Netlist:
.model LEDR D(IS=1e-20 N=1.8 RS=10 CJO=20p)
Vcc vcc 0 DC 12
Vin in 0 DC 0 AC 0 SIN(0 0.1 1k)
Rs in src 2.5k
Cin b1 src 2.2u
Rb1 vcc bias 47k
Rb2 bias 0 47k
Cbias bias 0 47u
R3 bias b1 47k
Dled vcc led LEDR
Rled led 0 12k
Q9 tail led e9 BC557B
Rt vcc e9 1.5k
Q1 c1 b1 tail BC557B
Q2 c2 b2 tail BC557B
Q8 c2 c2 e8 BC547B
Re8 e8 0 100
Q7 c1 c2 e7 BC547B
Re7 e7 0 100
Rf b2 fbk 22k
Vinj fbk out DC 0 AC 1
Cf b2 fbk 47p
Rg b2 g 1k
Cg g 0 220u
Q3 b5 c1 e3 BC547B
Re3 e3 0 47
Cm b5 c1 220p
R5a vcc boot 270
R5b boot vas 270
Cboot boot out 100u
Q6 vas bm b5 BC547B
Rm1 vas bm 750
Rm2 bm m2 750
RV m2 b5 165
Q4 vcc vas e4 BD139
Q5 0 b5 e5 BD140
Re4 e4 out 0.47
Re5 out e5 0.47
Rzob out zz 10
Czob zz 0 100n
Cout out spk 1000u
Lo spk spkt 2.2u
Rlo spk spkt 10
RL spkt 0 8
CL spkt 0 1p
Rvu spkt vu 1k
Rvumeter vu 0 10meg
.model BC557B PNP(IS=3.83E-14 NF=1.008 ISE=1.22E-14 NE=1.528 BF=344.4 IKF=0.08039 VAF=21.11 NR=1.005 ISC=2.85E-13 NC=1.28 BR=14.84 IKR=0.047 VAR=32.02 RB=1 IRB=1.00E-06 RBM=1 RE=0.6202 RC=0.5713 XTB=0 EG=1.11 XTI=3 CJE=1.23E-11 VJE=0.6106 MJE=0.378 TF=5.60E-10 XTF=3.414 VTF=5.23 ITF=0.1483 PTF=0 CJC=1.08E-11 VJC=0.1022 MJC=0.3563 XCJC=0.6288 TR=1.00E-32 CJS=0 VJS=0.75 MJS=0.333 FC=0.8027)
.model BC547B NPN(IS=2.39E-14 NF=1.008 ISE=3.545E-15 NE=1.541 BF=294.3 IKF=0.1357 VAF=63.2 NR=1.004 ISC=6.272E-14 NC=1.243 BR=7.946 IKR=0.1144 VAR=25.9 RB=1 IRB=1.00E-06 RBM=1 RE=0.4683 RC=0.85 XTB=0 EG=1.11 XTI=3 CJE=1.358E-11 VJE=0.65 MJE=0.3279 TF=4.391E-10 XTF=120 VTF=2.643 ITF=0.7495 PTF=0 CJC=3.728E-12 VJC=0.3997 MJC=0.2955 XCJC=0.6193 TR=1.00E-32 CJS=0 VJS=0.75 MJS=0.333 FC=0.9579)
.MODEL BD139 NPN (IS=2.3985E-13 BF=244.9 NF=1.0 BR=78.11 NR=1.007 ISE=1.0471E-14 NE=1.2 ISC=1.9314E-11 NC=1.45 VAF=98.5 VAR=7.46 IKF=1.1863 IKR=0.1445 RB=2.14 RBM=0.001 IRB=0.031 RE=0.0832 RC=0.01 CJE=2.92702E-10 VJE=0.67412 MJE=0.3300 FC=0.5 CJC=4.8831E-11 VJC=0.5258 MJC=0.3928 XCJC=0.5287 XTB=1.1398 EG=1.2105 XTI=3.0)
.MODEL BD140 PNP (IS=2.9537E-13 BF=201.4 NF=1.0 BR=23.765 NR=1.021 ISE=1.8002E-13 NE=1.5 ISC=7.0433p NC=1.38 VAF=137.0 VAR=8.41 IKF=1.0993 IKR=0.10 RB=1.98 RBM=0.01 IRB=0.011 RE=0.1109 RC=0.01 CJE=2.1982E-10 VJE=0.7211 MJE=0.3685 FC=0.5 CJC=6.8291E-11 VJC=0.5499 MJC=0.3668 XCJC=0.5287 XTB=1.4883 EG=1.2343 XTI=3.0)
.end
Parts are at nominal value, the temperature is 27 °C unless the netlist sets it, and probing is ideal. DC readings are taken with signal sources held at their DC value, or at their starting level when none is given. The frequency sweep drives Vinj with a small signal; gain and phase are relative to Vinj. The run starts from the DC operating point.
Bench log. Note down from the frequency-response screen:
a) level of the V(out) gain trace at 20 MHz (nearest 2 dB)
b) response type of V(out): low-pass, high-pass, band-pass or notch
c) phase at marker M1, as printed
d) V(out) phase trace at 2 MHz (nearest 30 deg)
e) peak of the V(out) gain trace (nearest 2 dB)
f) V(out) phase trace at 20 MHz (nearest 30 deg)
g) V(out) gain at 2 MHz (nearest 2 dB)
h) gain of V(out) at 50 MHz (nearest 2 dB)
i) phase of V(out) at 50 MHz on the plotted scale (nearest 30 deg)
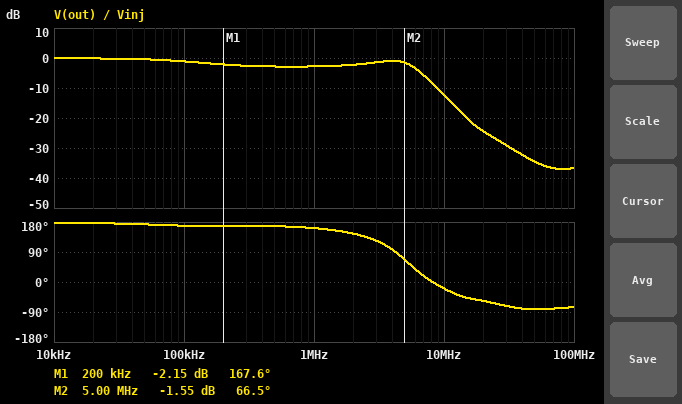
-24 dB
low-pass
167.6 deg
150 deg
0 dB
-60 deg
-2 dB
-34 dB
-90 deg
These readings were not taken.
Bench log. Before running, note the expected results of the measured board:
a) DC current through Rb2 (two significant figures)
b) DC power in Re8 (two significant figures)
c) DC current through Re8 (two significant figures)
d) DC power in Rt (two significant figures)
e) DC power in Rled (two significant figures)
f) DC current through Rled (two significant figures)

130 µA
15 µW
380 µA
970 µW
8.6 mW
850 µA
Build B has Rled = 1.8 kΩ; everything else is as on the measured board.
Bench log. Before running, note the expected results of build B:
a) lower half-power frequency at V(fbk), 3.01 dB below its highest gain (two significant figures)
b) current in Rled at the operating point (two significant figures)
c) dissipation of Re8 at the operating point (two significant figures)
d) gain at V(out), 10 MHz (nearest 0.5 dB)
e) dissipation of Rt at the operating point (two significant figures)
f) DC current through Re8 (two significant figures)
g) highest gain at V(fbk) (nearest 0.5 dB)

3.8 MHz
5.6 mA
18 µW
-11.5 dB
1.2 mW
430 µA
4.5 dB
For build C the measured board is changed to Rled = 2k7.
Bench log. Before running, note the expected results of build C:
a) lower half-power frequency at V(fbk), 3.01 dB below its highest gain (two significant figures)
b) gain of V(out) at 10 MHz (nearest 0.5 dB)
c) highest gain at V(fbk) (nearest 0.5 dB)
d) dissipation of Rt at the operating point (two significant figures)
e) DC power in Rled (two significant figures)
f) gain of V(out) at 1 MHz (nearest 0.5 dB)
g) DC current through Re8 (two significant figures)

3.8 MHz
-11.5 dB
4.5 dB
1.1 mW
38 mW
-2.5 dB
410 µA
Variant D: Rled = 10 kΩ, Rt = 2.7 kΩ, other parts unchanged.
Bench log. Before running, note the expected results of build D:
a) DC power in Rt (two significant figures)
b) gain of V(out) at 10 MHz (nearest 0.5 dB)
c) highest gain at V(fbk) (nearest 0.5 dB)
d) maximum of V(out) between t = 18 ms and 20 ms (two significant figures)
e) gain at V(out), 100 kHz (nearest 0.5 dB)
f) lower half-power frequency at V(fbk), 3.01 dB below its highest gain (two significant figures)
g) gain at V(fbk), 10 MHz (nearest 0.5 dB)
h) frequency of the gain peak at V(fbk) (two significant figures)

560 µW
-17.0 dB
2.5 dB
8.2 V
-2.0 dB
2.8 MHz
1.0 dB
5.3 MHz
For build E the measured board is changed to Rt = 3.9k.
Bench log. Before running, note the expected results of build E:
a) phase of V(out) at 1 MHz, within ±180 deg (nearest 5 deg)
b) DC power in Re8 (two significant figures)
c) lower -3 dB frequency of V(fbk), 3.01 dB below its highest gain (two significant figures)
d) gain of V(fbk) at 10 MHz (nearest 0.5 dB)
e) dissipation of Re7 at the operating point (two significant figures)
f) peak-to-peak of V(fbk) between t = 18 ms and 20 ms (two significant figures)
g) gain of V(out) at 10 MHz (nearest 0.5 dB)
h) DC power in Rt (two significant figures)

150 deg
1.9 µW
2.3 MHz
0.5 dB
2.0 µW
4.3 V
-21.0 dB
390 µW
